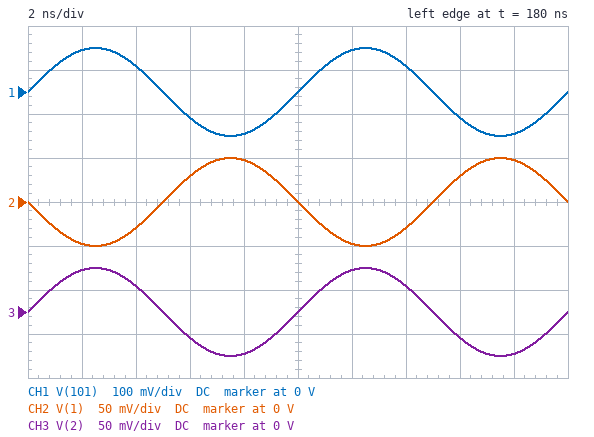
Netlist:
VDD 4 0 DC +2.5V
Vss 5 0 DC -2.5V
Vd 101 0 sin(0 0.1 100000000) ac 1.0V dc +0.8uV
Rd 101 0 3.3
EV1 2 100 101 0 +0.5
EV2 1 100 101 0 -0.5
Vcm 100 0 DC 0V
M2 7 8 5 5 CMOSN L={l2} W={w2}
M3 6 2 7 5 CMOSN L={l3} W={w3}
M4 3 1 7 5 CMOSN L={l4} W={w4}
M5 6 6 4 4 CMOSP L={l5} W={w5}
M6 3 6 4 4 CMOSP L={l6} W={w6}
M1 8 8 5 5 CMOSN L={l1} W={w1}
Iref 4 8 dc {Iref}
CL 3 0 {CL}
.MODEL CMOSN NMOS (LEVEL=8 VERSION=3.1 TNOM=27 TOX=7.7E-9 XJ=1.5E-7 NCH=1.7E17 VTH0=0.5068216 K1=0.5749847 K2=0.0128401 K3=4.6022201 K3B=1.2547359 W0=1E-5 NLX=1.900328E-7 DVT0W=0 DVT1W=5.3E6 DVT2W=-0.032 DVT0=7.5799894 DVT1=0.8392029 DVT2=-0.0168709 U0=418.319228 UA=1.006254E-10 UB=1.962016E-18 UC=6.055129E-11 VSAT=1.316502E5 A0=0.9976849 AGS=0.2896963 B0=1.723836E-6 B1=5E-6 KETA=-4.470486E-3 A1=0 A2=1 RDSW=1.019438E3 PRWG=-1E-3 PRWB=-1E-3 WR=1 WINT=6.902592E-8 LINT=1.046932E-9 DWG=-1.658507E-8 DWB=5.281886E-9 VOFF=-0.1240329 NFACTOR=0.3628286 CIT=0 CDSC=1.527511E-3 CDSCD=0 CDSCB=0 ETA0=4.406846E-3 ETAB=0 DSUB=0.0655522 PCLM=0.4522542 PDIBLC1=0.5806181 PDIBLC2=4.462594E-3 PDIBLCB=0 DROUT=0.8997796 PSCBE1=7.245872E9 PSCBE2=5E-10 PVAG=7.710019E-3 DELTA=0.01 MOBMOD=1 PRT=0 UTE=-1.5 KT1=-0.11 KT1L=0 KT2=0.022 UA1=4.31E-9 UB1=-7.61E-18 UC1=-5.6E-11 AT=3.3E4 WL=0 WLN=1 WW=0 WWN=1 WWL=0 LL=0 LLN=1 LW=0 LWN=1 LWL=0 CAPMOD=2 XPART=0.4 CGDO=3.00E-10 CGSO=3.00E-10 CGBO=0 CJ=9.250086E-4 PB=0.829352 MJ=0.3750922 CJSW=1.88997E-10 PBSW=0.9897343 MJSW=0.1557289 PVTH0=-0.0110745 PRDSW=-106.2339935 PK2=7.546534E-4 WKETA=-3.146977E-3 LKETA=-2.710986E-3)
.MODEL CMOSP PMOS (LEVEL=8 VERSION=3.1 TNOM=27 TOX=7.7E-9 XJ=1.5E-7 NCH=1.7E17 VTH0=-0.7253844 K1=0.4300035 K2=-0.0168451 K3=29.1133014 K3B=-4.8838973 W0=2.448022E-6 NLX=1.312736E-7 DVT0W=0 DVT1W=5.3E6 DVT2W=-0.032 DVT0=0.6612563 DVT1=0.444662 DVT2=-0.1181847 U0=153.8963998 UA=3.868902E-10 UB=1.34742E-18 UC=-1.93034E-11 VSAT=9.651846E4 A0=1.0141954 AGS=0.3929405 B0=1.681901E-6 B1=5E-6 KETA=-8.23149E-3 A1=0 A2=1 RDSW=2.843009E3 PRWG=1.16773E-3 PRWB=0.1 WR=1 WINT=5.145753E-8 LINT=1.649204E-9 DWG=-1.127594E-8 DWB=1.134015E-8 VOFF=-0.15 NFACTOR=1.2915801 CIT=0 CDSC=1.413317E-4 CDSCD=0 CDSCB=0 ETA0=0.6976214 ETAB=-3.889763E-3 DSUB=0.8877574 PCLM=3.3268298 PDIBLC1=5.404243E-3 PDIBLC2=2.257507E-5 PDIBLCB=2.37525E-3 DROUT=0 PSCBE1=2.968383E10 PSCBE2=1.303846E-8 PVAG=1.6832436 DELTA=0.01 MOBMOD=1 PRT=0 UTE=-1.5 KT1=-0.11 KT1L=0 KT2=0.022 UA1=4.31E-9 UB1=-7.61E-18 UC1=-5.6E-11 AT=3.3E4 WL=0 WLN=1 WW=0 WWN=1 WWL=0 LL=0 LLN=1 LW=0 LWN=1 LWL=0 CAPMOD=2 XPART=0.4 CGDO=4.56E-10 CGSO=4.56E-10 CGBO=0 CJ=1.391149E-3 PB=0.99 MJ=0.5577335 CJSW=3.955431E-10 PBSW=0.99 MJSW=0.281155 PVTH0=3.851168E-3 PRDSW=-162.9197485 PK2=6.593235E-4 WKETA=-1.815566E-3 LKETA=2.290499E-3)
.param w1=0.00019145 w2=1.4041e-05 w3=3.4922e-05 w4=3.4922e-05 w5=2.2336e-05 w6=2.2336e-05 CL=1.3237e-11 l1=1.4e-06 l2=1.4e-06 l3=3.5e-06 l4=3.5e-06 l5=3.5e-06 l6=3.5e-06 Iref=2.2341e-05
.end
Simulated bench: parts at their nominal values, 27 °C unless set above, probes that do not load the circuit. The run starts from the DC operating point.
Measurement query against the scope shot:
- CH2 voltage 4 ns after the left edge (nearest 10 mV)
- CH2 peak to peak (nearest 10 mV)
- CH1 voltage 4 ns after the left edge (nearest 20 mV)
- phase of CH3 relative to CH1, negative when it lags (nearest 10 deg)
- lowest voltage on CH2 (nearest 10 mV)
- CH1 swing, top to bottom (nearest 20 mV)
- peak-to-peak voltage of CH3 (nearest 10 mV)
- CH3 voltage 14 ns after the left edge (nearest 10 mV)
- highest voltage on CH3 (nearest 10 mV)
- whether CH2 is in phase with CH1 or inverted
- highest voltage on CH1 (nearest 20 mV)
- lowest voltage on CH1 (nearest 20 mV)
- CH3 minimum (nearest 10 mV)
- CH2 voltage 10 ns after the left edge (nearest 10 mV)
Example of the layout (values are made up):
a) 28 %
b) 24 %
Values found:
a) -30 mV
b) 100 mV
c) 60 mV
d) 0 deg
e) -50 mV
f) 200 mV
g) 100 mV
h) 30 mV
i) 50 mV
j) inverted
k) 100 mV
l) -100 mV
m) -50 mV
n) 0 V
